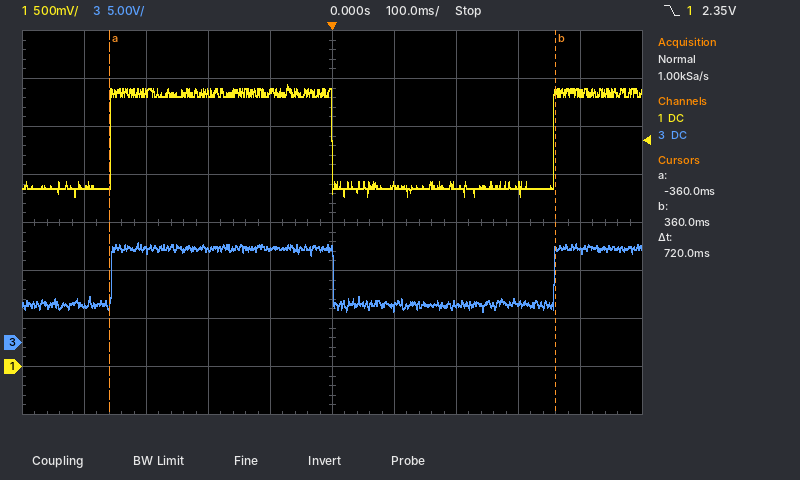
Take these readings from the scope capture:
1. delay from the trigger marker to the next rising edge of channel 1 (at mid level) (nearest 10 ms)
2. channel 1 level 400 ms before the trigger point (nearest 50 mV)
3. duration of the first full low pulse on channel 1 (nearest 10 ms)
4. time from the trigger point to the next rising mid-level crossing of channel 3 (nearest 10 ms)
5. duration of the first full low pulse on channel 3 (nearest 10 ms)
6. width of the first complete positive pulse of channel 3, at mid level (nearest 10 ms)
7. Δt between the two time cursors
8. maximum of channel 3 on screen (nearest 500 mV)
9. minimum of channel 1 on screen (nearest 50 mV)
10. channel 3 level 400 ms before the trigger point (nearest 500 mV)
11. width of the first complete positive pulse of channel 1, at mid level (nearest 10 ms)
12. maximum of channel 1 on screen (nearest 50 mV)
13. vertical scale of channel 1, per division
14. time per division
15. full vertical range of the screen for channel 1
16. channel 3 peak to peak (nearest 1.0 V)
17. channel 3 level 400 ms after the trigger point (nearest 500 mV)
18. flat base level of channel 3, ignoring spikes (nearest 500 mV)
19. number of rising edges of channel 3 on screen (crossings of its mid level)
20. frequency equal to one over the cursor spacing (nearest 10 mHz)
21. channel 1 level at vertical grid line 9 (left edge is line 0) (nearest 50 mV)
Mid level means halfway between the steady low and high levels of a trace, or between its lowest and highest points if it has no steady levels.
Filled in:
360 ms
1.85 V
360 ms
360 ms
360 ms
360 ms
720 ms
10.5 V
1.75 V
4.0 V
360 ms
2.95 V
500 mV
100 ms
4 V
7.0 V
9.5 V
4.0 V
2
1.39 Hz
2.85 V
